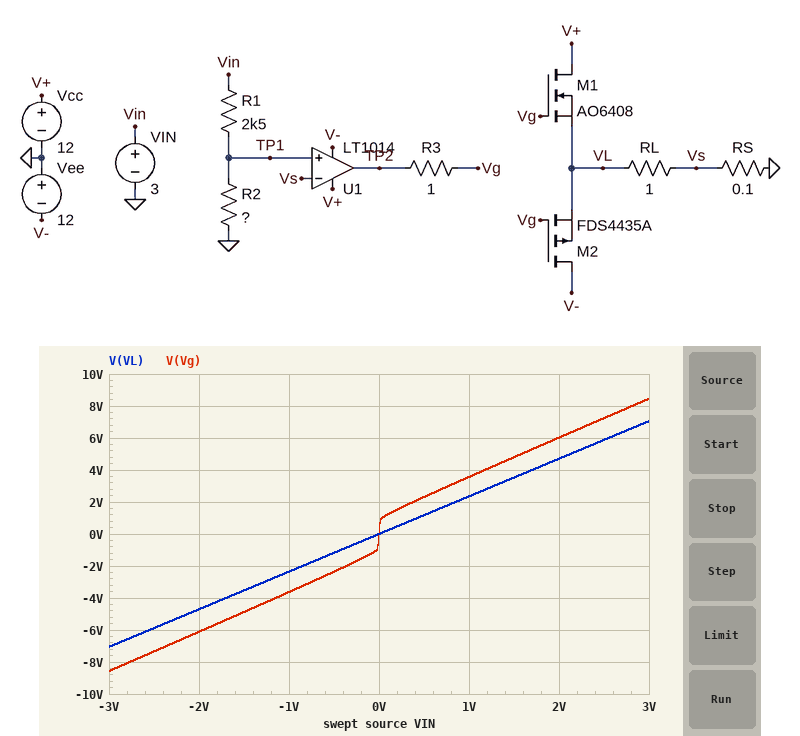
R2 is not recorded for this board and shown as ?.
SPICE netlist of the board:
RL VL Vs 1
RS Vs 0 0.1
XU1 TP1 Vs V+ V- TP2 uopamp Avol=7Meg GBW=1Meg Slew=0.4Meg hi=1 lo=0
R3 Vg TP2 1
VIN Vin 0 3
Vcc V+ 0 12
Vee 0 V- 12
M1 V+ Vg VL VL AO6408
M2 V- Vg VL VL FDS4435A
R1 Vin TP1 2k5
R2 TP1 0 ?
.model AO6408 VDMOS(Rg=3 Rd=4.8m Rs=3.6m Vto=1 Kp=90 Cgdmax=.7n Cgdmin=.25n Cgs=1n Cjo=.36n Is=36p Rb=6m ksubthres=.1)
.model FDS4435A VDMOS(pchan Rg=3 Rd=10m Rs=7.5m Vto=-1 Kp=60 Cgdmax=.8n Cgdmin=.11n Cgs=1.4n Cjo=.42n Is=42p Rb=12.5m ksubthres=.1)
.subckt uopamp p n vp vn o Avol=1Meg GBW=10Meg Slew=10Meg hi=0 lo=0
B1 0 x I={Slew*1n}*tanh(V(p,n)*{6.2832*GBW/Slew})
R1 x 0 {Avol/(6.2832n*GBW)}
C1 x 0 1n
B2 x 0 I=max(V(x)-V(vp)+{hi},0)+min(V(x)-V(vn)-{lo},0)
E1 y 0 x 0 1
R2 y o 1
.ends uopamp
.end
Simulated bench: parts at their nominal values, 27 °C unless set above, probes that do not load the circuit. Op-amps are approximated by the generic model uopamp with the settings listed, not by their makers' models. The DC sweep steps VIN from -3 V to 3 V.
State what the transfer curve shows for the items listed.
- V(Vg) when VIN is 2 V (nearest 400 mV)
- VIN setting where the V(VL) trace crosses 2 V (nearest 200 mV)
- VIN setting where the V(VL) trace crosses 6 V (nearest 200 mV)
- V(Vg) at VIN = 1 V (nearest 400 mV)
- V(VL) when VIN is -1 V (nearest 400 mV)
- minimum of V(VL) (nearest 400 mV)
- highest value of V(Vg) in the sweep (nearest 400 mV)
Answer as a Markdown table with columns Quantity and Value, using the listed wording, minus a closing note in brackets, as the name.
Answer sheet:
| Quantity | Value |
|---|---|
| V(Vg) when VIN is 2 V | 6.0 V |
| VIN setting where the V(VL) trace crosses 2 V | 800 mV |
| VIN setting where the V(VL) trace crosses 6 V | 2.6 V |
| V(Vg) at VIN = 1 V | 3.6 V |
| V(VL) when VIN is -1 V | -2.4 V |
| minimum of V(VL) | -7.2 V |
| highest value of V(Vg) in the sweep | 8.4 V |
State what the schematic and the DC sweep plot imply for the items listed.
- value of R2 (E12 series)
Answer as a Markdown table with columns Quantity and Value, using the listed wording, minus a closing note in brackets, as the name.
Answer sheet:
| Quantity | Value |
|---|---|
| value of R2 | 680 Ω |
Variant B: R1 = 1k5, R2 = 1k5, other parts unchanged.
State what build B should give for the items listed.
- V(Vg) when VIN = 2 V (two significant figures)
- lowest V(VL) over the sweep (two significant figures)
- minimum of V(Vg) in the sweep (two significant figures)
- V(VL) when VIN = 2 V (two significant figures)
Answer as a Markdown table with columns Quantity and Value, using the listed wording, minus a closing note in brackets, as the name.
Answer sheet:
| Quantity | Value |
|---|---|
| V(Vg) when VIN = 2 V | 11 V |
| lowest V(VL) over the sweep | -10 V |
| minimum of V(Vg) in the sweep | -12 V |
| V(VL) when VIN = 2 V | 9.5 V |
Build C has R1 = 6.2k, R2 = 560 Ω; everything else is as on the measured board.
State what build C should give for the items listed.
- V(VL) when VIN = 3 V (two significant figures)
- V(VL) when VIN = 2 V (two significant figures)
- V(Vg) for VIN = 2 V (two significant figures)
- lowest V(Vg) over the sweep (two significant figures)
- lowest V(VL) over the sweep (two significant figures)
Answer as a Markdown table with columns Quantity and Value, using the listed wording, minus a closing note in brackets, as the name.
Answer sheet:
| Quantity | Value |
|---|---|
| V(VL) when VIN = 3 V | 2.7 V |
| V(VL) when VIN = 2 V | 1.8 V |
| V(Vg) for VIN = 2 V | 3.0 V |
| lowest V(Vg) over the sweep | -4.0 V |
| lowest V(VL) over the sweep | -2.7 V |
